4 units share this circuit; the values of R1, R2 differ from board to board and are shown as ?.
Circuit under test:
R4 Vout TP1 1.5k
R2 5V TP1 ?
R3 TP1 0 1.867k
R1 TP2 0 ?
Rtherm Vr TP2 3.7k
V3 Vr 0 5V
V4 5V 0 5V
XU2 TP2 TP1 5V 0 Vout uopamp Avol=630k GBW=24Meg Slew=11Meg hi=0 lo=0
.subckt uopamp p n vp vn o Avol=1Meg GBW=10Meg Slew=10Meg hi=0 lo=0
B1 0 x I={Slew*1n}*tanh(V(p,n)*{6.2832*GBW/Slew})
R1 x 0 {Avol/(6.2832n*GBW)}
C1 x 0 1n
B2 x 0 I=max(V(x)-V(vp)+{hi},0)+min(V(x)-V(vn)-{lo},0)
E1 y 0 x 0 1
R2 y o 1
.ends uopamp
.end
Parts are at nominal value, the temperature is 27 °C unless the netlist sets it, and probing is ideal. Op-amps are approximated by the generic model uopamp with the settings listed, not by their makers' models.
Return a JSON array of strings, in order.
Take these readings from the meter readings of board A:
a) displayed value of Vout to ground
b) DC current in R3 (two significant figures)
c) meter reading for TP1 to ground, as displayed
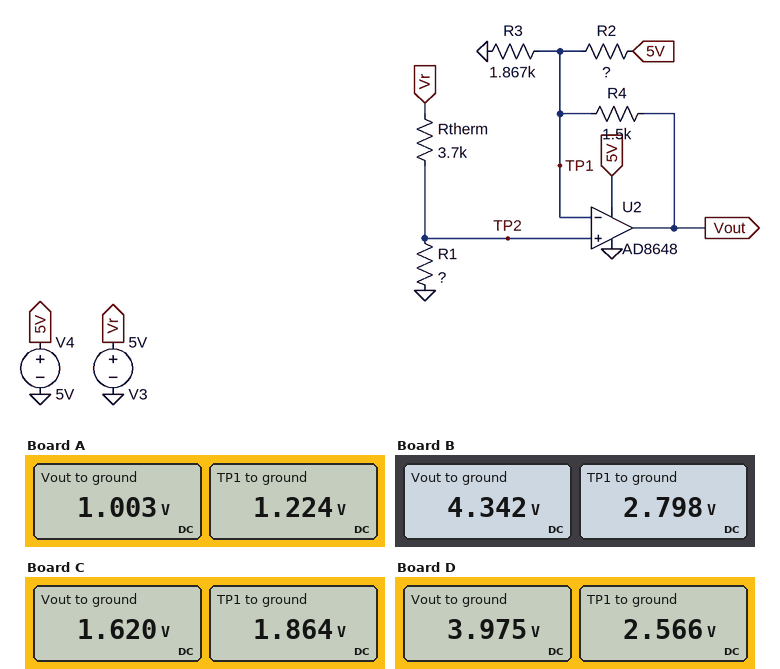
["1.003 V", "660 µA", "1.224 V"]
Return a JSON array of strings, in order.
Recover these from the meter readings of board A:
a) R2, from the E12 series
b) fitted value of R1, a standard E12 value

["4.7 kΩ", "1.2 kΩ"]
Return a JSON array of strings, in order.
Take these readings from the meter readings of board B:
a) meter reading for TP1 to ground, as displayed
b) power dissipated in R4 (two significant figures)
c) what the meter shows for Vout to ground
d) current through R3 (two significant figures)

["2.798 V", "1.6 mW", "4.342 V", "1.5 mA"]
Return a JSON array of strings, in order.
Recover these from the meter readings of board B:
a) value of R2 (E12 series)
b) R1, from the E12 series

["4.7 kΩ", "4.7 kΩ"]
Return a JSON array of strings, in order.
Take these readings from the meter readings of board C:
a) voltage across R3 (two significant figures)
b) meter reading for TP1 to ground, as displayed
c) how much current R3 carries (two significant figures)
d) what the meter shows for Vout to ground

["1.9 V", "1.864 V", "1.0 mA", "1.620 V"]
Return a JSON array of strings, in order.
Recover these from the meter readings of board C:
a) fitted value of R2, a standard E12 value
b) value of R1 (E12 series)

["2.7 kΩ", "2.2 kΩ"]
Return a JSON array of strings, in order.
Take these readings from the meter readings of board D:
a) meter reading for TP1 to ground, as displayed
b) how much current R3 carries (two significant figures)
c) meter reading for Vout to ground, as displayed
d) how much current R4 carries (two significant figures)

["2.566 V", "1.4 mA", "3.975 V", "940 µA"]
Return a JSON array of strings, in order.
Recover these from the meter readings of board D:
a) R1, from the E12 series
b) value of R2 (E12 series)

["3.9 kΩ", "5.6 kΩ"]
